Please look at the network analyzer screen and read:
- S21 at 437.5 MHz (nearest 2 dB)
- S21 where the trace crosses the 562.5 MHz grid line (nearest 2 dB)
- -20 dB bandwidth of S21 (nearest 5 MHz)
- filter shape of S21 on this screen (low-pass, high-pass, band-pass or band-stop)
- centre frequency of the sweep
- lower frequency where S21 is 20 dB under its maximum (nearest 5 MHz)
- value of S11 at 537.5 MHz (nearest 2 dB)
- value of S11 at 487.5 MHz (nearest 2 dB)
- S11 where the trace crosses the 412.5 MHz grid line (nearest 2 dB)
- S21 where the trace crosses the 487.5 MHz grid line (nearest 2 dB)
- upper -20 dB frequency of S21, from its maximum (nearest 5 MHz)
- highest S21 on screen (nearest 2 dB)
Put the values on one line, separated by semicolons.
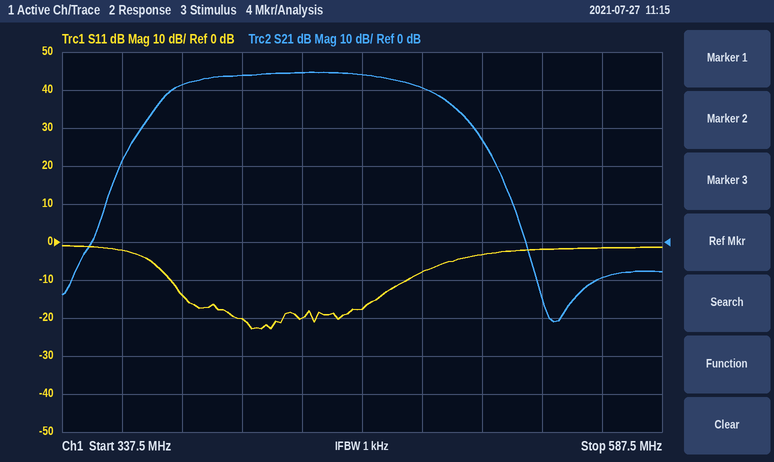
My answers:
44 dB; -10 dB; 150 MHz; band-pass; 462.5 MHz; 365 MHz; -2 dB; -8 dB; -20 dB; 40 dB; 515 MHz; 44 dB
